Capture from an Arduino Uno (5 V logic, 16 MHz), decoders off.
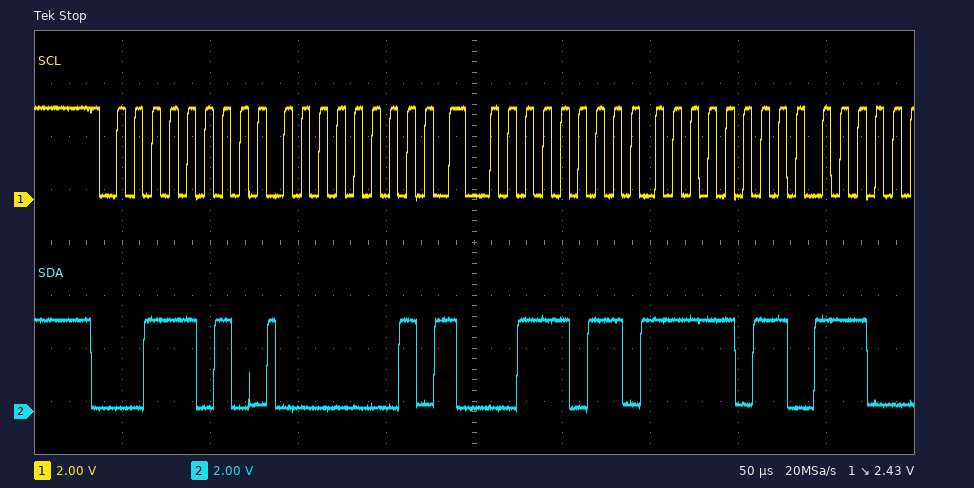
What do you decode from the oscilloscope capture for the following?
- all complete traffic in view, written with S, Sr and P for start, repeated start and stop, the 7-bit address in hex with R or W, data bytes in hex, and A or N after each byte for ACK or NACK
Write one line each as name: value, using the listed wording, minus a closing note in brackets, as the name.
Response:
all complete traffic in view, written with S, Sr and P for start, repeated start and stop, the 7-bit address in hex with R or W, data bytes in hex, and A or N after each byte for ACK or NACK: S 1DW A 01 A Sr 1DR A FB A
